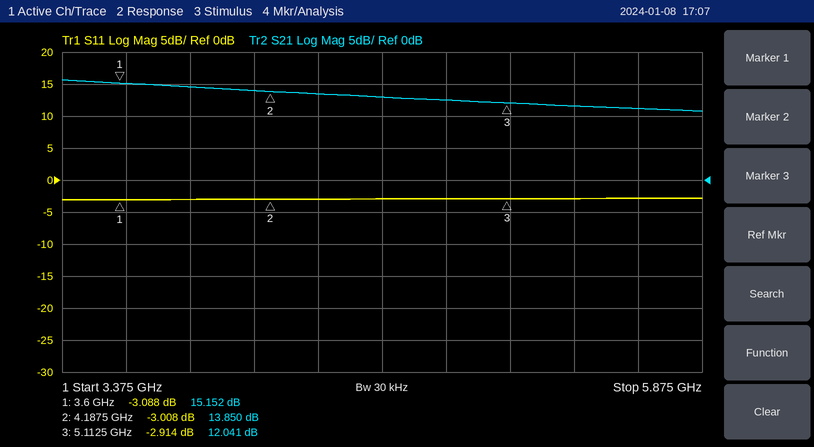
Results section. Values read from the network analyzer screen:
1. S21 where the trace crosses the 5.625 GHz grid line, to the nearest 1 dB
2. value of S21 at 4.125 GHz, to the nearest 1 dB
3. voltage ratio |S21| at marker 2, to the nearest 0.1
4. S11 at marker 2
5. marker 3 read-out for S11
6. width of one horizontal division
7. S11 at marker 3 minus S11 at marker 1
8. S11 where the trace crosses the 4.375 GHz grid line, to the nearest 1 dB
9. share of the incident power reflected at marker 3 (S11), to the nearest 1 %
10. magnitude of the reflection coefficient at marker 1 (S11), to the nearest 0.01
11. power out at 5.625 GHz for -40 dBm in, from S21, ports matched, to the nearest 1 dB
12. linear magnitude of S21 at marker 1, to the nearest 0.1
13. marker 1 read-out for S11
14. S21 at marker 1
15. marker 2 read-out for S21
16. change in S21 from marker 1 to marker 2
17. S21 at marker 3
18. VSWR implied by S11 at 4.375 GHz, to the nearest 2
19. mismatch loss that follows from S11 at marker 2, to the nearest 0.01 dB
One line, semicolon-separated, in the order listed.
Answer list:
11 dB; 14 dB; 4.9; -3.008 dB; -2.914 dB; 250 MHz; 0.174 dB; -3 dB; 51 %; 0.70; -29 dBm; 5.7; -3.088 dB; 15.152 dB; 13.850 dB; -1.302 dB; 12.041 dB; 6; 3.01 dB
